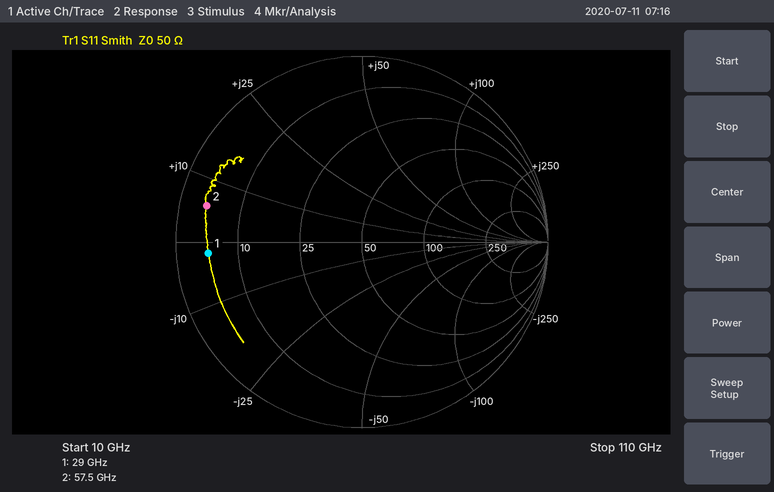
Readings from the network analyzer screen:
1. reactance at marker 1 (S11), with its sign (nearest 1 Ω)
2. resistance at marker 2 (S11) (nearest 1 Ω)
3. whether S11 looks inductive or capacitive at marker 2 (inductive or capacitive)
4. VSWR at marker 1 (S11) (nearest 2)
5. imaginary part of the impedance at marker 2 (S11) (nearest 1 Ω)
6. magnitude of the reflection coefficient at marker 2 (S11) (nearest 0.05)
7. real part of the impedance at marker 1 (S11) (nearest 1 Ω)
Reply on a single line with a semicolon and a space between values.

-2 Ω; 4 Ω; inductive; 10; +6 Ω; 0.85; 5 Ω
